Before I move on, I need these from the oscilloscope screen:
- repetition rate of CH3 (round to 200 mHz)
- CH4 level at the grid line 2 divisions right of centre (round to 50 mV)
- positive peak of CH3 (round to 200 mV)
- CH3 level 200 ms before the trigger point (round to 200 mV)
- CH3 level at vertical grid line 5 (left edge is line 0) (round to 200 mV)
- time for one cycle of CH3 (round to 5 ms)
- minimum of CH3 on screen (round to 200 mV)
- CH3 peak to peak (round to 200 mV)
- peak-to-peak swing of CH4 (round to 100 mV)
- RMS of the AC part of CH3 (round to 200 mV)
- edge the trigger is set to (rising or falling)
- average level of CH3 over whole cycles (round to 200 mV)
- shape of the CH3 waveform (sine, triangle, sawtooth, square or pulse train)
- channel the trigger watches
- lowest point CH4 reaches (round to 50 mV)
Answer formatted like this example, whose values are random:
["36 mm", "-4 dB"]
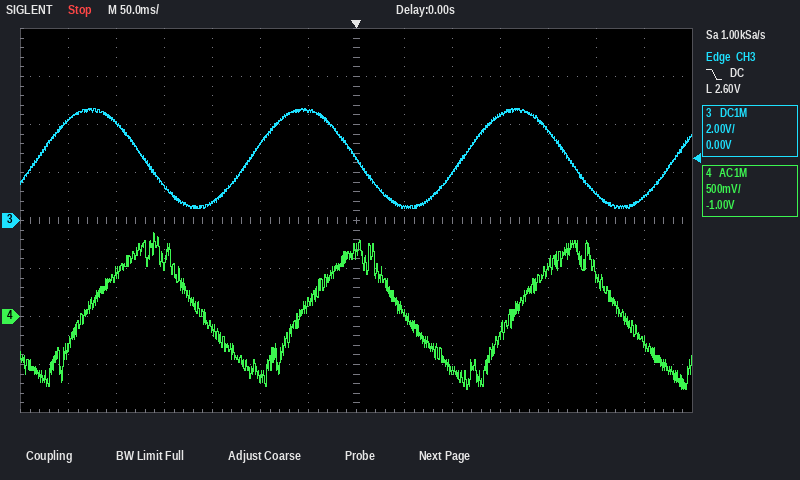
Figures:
["4.6 Hz", "-550 mV", "4.6 V", "1.4 V", "3.2 V", "220 ms", "400 mV", "4.2 V", "1.60 V", "1.4 V", "falling", "2.6 V", "sine", "CH3", "-750 mV"]
